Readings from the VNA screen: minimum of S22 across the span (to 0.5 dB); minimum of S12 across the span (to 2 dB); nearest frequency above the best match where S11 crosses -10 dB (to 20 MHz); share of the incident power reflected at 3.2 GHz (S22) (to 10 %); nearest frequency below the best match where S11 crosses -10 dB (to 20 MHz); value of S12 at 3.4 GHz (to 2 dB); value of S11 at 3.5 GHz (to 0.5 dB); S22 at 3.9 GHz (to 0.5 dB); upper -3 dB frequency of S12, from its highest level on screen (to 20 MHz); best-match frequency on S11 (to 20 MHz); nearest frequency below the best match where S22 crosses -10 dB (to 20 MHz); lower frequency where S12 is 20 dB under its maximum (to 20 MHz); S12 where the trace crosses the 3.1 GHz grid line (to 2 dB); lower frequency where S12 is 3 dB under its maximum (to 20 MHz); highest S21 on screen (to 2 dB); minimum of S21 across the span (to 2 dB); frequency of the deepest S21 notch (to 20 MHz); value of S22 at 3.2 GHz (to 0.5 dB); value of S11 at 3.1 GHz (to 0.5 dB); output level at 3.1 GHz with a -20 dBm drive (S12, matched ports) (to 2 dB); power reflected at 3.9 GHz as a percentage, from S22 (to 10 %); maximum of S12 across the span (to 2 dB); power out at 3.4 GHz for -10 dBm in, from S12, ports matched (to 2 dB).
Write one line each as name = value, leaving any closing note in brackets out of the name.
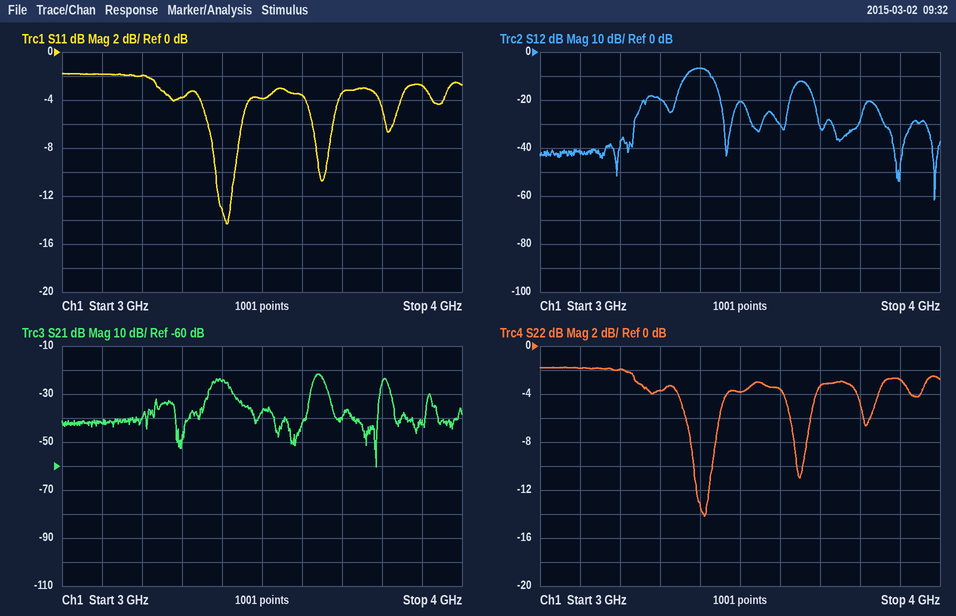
minimum of S22 across the span = -14.0 dB
minimum of S12 across the span = -62 dB
nearest frequency above the best match where S11 crosses -10 dB = 3.44 GHz
share of the incident power reflected at 3.2 GHz (S22) = 60 %
nearest frequency below the best match where S11 crosses -10 dB = 3.38 GHz
value of S12 at 3.4 GHz = -6 dB
value of S11 at 3.5 GHz = -4.0 dB
S22 at 3.9 GHz = -3.0 dB
upper -3 dB frequency of S12, from its highest level on screen = 3.42 GHz
best-match frequency on S11 = 3.42 GHz
nearest frequency below the best match where S22 crosses -10 dB = 3.38 GHz
lower frequency where S12 is 20 dB under its maximum = 3.24 GHz
S12 where the trace crosses the 3.1 GHz grid line = -42 dB
lower frequency where S12 is 3 dB under its maximum = 3.36 GHz
highest S21 on screen = -22 dB
minimum of S21 across the span = -60 dB
frequency of the deepest S21 notch = 3.78 GHz
value of S22 at 3.2 GHz = -2.0 dB
value of S11 at 3.1 GHz = -2.0 dB
output level at 3.1 GHz with a -20 dBm drive (S12, matched ports) = -62 dBm
power reflected at 3.9 GHz as a percentage, from S22 = 50 %
maximum of S12 across the span = -6 dB
power out at 3.4 GHz for -10 dBm in, from S12, ports matched = -16 dBm
